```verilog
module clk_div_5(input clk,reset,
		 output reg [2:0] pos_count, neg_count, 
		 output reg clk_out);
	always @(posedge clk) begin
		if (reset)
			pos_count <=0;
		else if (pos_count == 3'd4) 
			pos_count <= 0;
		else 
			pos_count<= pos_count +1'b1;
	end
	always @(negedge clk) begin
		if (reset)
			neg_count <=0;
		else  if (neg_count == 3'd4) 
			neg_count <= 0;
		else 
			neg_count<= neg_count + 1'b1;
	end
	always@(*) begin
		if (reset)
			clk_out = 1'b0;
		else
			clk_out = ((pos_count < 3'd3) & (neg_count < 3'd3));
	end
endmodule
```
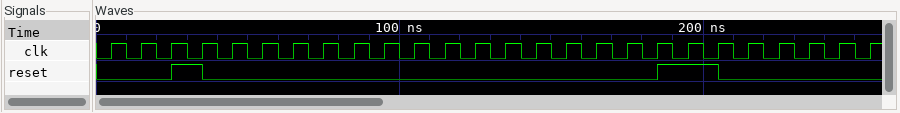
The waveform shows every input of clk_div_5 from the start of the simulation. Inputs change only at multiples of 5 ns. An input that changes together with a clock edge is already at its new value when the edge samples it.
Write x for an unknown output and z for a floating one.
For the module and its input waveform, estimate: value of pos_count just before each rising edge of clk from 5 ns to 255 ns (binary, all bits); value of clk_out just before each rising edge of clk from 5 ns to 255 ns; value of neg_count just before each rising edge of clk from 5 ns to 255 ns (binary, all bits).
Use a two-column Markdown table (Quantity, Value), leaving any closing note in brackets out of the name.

| Quantity | Value |
|---|---|
| value of pos_count just before each rising edge of clk from 5 ns to 255 ns | x, x, x, 000, 001, 010, 011, 100, 000, 001, 010, 011, 100, 000, 001, 010, 011, 100, 000, 000, 000, 001, 010, 011, 100, 000 |
| value of clk_out just before each rising edge of clk from 5 ns to 255 ns | x x x 0 1 1 0 0 1 1 1 0 0 1 1 1 0 0 1 0 0 1 1 0 0 1 |
| value of neg_count just before each rising edge of clk from 5 ns to 255 ns | x, x, x, 000, 001, 010, 011, 100, 000, 001, 010, 011, 100, 000, 001, 010, 011, 100, 000, 000, 000, 001, 010, 011, 100, 000 |
